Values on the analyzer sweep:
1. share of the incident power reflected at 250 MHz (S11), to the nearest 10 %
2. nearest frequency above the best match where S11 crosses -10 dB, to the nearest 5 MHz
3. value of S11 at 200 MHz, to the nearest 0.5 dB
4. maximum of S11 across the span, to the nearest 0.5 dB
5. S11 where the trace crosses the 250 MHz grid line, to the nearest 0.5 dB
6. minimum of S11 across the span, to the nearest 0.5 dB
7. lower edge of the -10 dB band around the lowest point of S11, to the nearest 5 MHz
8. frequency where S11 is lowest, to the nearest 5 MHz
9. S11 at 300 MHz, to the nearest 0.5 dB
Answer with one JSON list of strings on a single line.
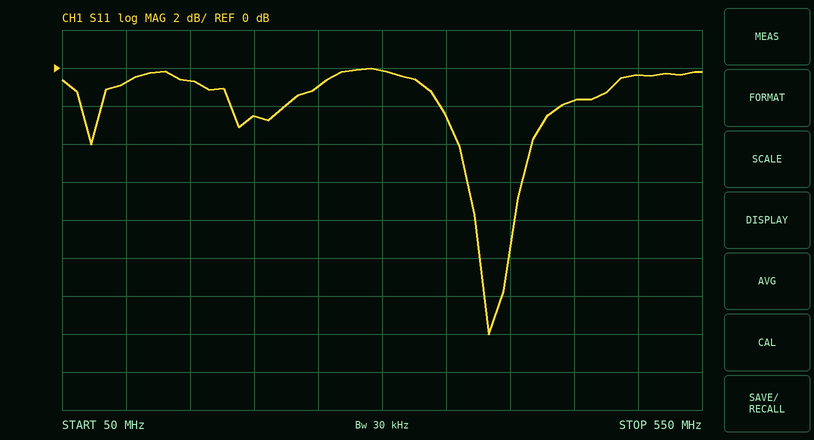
["80 %", "400 MHz", "-2.5 dB", "0.0 dB", "-1.0 dB", "-14.0 dB", "375 MHz", "385 MHz", "0.0 dB"]
